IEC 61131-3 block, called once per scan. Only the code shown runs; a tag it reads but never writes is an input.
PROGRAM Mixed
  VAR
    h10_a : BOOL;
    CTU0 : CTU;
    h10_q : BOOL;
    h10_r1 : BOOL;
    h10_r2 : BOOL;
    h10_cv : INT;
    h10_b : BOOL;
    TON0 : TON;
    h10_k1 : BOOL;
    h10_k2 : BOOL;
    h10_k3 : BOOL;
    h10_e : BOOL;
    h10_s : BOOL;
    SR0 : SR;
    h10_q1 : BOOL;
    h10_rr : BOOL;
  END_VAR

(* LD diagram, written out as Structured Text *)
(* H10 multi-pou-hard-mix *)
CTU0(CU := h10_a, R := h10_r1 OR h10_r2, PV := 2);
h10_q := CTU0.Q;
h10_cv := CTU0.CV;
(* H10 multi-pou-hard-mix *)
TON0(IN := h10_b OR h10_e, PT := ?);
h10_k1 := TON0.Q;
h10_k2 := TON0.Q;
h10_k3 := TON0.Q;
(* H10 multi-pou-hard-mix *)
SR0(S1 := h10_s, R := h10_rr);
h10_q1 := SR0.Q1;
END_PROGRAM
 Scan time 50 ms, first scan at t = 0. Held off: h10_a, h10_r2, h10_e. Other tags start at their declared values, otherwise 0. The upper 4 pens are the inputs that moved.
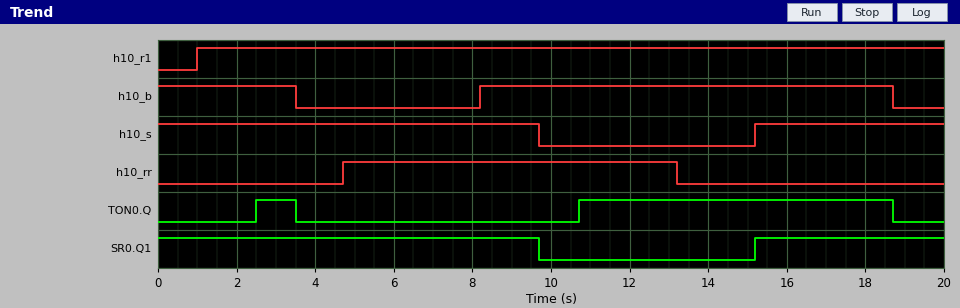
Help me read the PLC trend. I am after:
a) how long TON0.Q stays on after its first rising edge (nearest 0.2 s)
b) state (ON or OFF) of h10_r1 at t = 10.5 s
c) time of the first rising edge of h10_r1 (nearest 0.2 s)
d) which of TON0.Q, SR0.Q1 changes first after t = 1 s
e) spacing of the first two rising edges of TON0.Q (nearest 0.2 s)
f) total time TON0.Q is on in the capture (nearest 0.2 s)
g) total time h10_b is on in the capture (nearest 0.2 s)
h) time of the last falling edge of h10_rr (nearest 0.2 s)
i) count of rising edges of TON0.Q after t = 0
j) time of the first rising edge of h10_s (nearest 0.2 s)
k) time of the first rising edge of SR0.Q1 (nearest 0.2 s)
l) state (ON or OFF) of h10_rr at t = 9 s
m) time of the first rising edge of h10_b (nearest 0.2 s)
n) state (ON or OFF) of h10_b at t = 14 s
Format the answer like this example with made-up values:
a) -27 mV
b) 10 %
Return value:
a) 1.0 s
b) ON
c) 1.0 s
d) TON0.Q
e) 8.2 s
f) 9.0 s
g) 14.0 s
h) 13.2 s
i) 2
j) 15.2 s
k) 15.2 s
l) ON
m) 8.2 s
n) ON
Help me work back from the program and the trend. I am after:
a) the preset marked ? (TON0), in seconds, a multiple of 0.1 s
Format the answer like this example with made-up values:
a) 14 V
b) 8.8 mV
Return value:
a) 2.5 s
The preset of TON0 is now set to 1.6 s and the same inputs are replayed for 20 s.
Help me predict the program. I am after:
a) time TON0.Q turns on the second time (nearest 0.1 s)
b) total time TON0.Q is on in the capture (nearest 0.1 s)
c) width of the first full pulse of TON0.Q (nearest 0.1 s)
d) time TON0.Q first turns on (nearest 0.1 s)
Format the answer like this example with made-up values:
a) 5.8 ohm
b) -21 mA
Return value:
a) 9.8 s
b) 10.8 s
c) 1.9 s
d) 1.6 s
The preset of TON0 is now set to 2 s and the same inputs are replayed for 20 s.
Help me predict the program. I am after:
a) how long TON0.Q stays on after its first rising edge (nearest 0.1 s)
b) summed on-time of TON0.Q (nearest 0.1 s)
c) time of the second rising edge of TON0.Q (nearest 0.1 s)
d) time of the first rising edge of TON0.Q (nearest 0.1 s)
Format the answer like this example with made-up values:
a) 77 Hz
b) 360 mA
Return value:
a) 1.5 s
b) 10.0 s
c) 10.2 s
d) 2.0 s
